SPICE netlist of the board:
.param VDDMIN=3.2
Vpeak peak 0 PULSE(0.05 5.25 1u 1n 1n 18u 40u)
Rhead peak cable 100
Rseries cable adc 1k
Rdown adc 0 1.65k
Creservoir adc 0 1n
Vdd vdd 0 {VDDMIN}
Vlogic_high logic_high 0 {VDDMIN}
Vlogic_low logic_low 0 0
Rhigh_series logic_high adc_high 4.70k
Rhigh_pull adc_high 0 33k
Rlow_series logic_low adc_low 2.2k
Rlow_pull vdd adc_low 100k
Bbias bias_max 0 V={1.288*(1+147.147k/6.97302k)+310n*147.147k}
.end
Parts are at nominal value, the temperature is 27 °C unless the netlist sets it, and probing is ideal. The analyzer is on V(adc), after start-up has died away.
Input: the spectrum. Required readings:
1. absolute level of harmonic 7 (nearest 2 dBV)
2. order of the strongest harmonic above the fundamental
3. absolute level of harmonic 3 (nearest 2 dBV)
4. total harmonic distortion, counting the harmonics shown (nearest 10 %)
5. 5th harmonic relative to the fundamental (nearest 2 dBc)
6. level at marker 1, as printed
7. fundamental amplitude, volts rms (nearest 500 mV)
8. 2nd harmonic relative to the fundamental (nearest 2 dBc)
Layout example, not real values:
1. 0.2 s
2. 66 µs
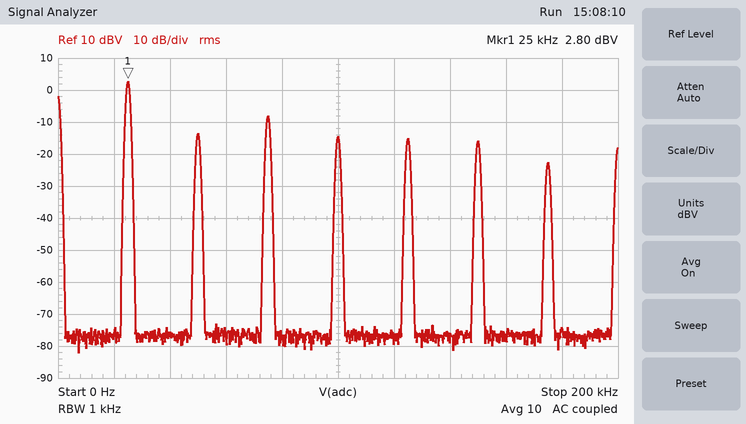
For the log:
1. -22 dBV
2. 3
3. -8 dBV
4. 40 %
5. -18 dBc
6. 2.80 dBV
7. 1.5 V
8. -16 dBc
